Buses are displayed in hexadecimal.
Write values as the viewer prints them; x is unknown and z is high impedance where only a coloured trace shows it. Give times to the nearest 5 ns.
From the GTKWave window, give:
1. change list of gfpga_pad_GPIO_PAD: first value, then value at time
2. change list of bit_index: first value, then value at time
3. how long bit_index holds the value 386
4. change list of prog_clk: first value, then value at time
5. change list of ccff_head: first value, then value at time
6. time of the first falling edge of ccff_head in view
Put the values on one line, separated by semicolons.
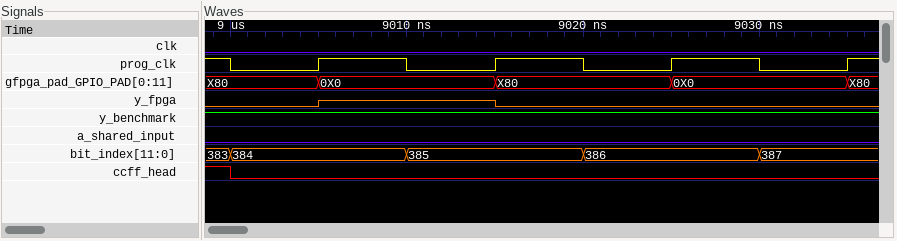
X80, 0X0 at 9005 ns, X80 at 9015 ns, 0X0 at 9025 ns, X80 at 9035 ns; 383, 384 at 9000 ns, 385 at 9010 ns, 386 at 9020 ns, 387 at 9030 ns; 10 ns; 1, 0 at 9000 ns, 1 at 9005 ns, 0 at 9010 ns, 1 at 9015 ns, 0 at 9020 ns, 1 at 9025 ns, 0 at 9030 ns, 1 at 9035 ns; 1, 0 at 9000 ns; 9000 ns
